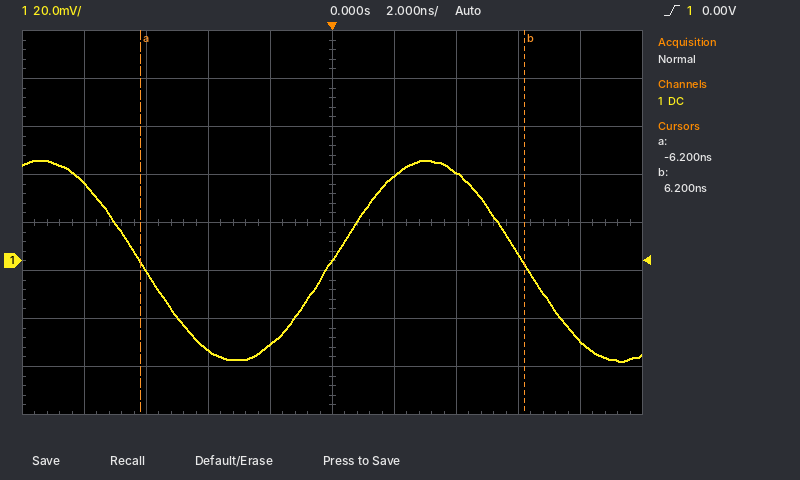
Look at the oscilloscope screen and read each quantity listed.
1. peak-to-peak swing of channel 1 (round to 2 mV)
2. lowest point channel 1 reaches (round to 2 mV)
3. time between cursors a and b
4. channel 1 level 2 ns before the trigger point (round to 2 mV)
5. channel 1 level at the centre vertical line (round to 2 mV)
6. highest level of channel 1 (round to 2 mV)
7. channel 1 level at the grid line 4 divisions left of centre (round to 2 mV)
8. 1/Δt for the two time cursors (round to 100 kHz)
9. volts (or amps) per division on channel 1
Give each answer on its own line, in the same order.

84 mV
-42 mV
12.4 ns
-34 mV
0 mV
42 mV
32 mV
80.6 MHz
20 mV
